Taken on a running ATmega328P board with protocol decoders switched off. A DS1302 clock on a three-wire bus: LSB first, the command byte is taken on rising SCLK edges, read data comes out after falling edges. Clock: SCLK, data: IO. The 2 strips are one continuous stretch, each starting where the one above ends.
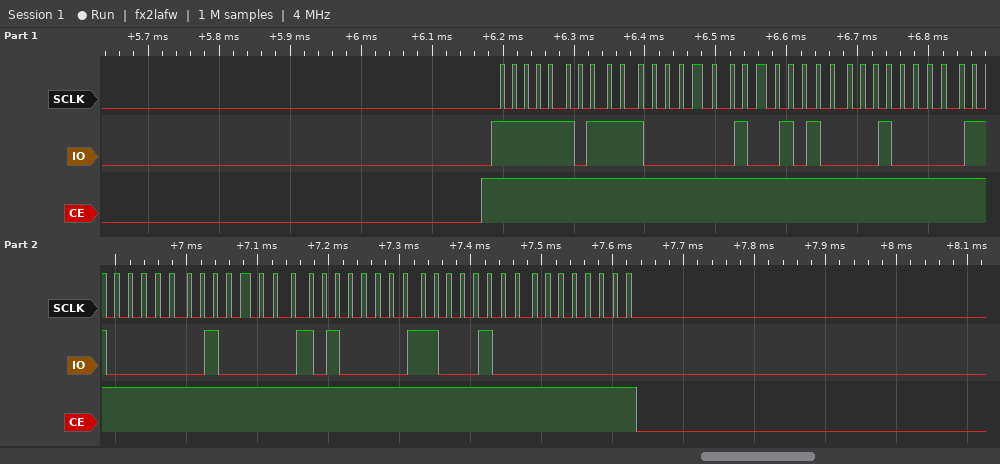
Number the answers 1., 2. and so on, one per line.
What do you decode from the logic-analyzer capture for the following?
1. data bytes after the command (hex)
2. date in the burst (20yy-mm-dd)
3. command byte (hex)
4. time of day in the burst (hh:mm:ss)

1. 07 52 08 06 04 05 23 00
2. 2023-04-06
3. 0xBF
4. 08:52:07
